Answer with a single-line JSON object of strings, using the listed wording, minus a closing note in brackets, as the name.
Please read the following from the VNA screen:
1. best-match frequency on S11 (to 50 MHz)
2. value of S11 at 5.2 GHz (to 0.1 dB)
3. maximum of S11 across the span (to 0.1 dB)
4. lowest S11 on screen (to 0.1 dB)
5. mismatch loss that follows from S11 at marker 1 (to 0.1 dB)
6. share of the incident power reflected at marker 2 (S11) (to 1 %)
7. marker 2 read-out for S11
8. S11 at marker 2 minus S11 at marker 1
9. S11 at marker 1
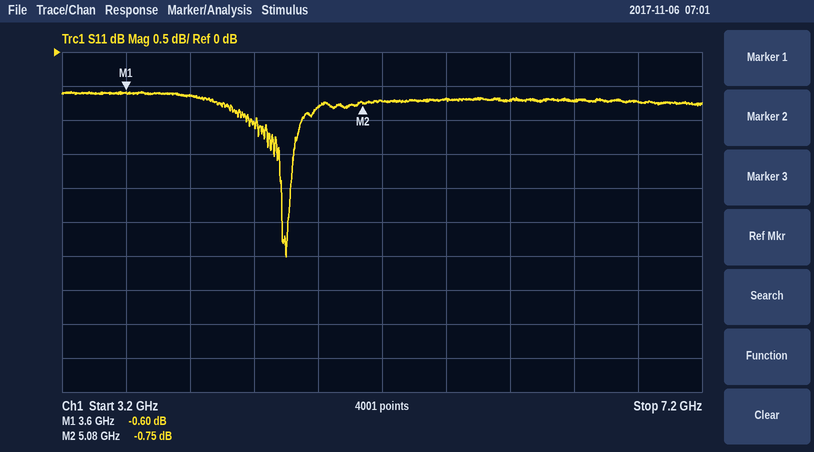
{"best-match frequency on S11": "4.60 GHz", "value of S11 at 5.2 GHz": "-0.7 dB", "maximum of S11 across the span": "-0.6 dB", "lowest S11 on screen": "-3.0 dB", "mismatch loss that follows from S11 at marker 1": "8.9 dB", "share of the incident power reflected at marker 2 (S11)": "84 %", "marker 2 read-out for S11": "-0.75 dB", "S11 at marker 2 minus S11 at marker 1": "-0.15 dB", "S11 at marker 1": "-0.60 dB"}
